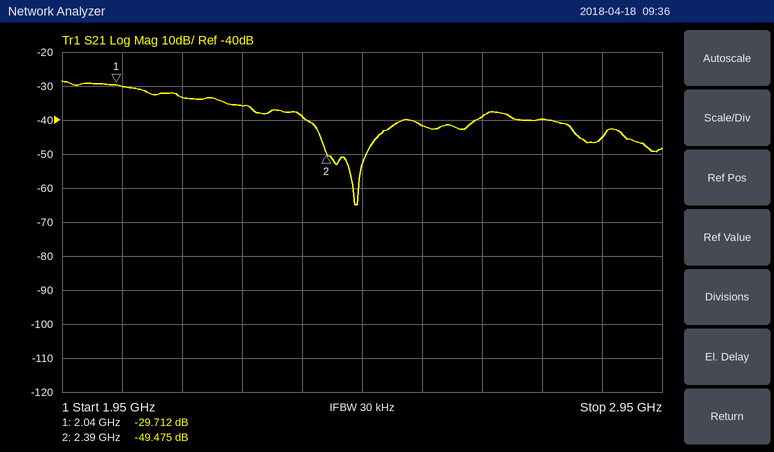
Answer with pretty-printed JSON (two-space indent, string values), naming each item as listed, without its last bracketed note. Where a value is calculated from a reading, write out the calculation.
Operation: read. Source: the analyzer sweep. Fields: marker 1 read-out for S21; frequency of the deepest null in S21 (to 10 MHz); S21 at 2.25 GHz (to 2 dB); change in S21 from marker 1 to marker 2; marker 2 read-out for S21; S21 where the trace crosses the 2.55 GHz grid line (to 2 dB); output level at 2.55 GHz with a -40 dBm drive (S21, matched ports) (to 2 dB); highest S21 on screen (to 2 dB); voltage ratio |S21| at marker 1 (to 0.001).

{
  "marker 1 read-out for S21": "-29.712 dB",
  "frequency of the deepest null in S21": "2.44 GHz",
  "S21 at 2.25 GHz": "-36 dB",
  "change in S21 from marker 1 to marker 2": "-49.475 − (-29.712) = -19.763 dB",
  "marker 2 read-out for S21": "-49.475 dB",
  "S21 where the trace crosses the 2.55 GHz grid line": "-42 dB",
  "output level at 2.55 GHz with a -40 dBm drive (S21, matched ports)": "-40 dBm + (-42 dB) = -82 dBm",
  "highest S21 on screen": "-28 dB",
  "voltage ratio |S21| at marker 1": "10^(-29.712/20) ≈ 0.033"
}
